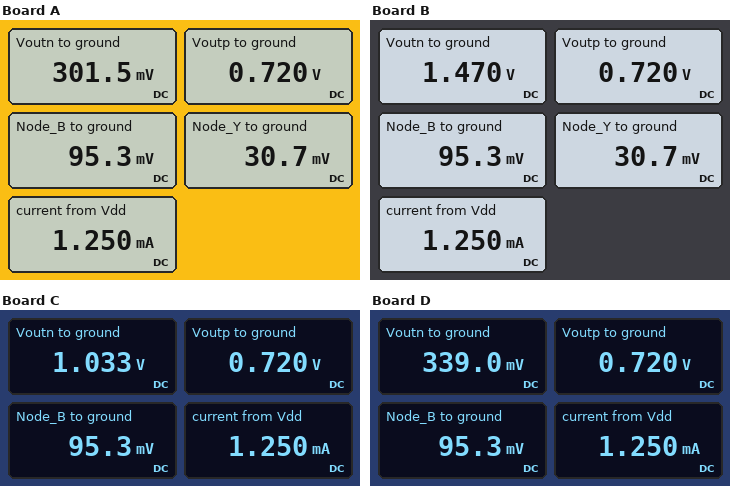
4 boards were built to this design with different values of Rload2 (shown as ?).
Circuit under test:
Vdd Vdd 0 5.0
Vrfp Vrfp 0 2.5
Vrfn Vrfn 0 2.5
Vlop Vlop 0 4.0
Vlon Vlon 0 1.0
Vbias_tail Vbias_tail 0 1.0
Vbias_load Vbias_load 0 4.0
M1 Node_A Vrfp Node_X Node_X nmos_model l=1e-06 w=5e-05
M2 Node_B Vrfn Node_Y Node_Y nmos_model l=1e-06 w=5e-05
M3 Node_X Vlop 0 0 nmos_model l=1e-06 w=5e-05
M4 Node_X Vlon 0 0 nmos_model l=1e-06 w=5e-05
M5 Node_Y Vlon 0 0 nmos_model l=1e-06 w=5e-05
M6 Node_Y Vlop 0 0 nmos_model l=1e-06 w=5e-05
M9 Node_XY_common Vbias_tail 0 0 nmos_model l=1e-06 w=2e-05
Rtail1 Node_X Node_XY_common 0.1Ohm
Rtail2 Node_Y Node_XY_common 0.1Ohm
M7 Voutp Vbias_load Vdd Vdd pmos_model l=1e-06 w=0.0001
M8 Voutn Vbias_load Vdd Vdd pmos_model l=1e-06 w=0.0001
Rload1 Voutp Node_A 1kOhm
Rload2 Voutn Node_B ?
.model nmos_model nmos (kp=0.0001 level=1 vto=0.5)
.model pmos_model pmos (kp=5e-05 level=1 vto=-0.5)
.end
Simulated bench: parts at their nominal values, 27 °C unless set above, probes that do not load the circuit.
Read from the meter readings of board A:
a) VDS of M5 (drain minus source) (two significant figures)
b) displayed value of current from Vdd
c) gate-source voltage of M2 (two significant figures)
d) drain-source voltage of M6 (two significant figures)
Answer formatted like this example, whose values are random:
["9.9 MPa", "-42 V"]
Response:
["31 mV", "1.250 mA", "2.5 V", "31 mV"]
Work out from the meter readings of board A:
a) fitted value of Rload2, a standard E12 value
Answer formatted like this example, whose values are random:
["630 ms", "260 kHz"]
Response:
["330 Ω"]
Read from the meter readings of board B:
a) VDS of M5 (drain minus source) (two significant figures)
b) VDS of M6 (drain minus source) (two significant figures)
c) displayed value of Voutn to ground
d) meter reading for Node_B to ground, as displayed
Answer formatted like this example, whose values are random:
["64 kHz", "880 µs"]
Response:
["31 mV", "31 mV", "1.470 V", "95.3 mV"]
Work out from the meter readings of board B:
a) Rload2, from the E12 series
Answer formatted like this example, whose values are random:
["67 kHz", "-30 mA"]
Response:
["2.2 kΩ"]
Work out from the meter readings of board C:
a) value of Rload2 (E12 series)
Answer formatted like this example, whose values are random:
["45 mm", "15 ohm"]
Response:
["1.5 kΩ"]
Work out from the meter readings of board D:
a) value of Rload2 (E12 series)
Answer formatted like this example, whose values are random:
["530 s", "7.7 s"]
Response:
["390 Ω"]
